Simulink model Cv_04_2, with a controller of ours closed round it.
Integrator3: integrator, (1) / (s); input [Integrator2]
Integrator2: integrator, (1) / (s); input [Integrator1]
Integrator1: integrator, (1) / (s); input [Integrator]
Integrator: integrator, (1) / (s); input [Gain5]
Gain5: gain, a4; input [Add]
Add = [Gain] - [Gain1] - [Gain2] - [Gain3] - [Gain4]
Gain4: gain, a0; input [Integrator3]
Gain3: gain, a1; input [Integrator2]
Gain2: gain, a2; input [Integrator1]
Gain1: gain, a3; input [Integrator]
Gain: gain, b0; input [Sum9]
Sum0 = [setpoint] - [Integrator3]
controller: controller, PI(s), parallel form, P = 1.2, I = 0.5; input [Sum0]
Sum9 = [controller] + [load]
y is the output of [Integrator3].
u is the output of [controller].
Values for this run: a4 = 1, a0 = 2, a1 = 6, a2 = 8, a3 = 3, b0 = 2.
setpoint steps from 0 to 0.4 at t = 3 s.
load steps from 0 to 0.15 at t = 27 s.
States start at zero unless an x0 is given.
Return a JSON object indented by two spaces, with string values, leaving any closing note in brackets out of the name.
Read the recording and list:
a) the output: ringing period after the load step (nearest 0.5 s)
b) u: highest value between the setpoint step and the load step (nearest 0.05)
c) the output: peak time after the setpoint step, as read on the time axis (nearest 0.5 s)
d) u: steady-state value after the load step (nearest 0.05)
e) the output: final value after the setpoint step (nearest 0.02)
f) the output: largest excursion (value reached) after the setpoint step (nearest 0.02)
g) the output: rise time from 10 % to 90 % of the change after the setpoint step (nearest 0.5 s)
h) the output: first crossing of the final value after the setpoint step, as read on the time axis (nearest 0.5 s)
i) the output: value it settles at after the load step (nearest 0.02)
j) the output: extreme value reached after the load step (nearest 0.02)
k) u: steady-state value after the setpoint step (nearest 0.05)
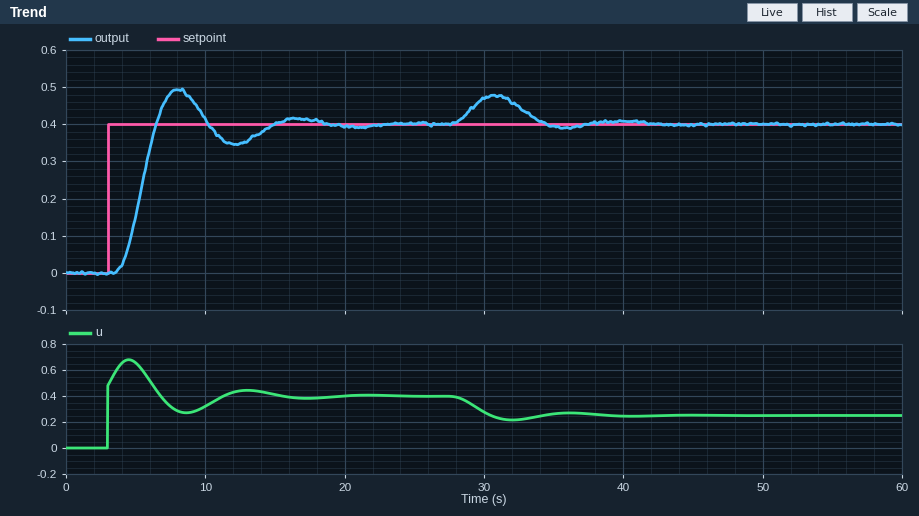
{
  "the output: ringing period after the load step": "9.0 s",
  "u: highest value between the setpoint step and the load step": "0.70",
  "the output: peak time after the setpoint step, as read on the time axis": "8.0 s",
  "u: steady-state value after the load step": "0.25",
  "the output: final value after the setpoint step": "0.40",
  "the output: largest excursion (value reached) after the setpoint step": "0.50",
  "the output: rise time from 10 % to 90 % of the change after the setpoint step": "2.0 s",
  "the output: first crossing of the final value after the setpoint step, as read on the time axis": "6.5 s",
  "the output: value it settles at after the load step": "0.40",
  "the output: extreme value reached after the load step": "0.48",
  "u: steady-state value after the setpoint step": "0.40"
}
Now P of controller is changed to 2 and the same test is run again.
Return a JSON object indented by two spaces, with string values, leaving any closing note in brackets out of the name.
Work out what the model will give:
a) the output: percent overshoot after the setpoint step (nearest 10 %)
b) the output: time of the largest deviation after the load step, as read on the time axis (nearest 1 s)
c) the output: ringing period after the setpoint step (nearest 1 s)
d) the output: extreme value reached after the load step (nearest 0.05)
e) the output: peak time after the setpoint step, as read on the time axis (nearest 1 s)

{
  "the output: percent overshoot after the setpoint step": "30 %",
  "the output: time of the largest deviation after the load step, as read on the time axis": "30 s",
  "the output: ringing period after the setpoint step": "7 s",
  "the output: extreme value reached after the load step": "0.45",
  "the output: peak time after the setpoint step, as read on the time axis": "7 s"
}
